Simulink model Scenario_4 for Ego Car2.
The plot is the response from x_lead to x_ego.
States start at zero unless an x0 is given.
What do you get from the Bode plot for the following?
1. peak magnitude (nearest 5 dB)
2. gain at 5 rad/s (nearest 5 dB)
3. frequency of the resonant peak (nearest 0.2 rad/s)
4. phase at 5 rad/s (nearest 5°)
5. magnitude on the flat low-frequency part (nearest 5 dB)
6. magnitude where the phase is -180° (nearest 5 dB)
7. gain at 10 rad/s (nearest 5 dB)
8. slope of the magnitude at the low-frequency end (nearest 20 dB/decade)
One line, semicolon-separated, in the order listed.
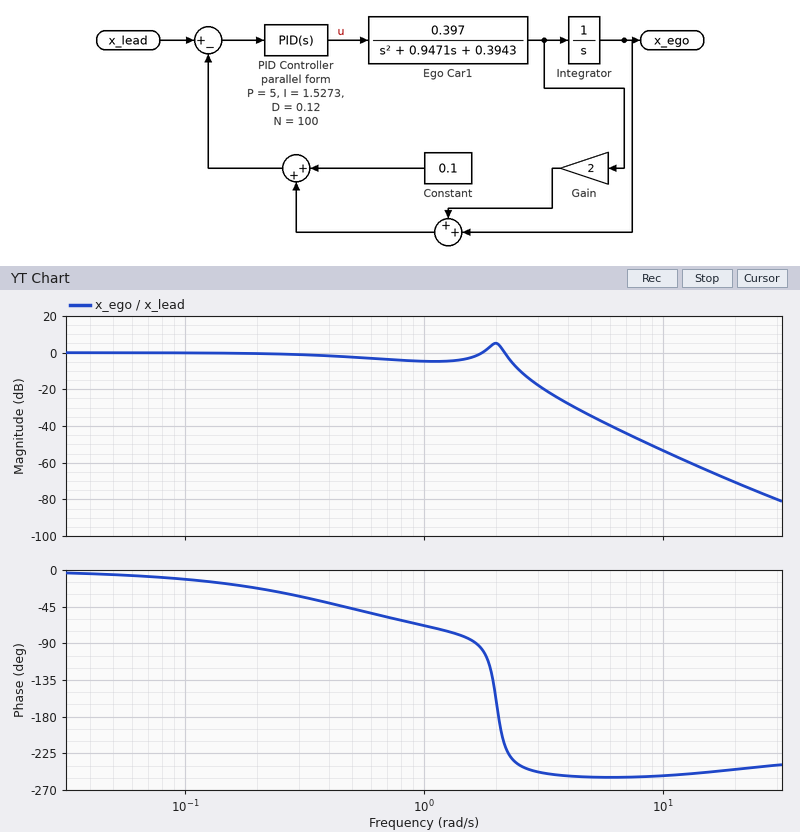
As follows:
5 dB; -35 dB; 2.0 rad/s; -255°; 0 dB; 5 dB; -55 dB; 0 dB/decade
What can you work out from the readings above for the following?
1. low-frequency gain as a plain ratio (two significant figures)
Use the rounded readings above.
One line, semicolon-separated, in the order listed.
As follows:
1.0
